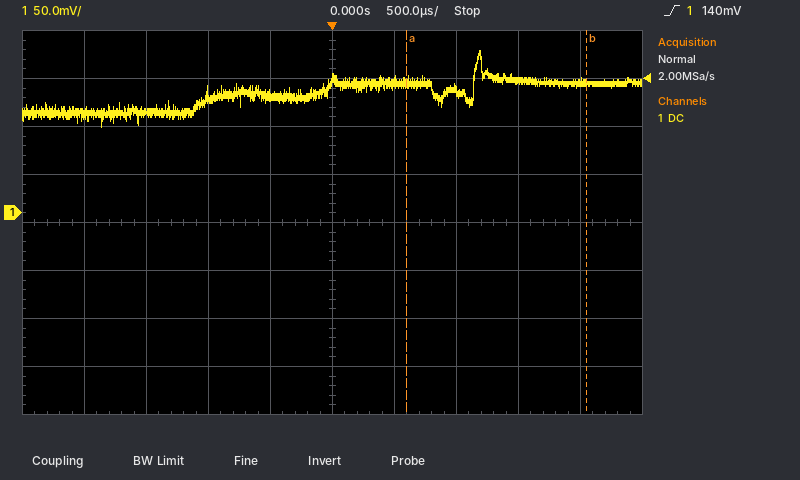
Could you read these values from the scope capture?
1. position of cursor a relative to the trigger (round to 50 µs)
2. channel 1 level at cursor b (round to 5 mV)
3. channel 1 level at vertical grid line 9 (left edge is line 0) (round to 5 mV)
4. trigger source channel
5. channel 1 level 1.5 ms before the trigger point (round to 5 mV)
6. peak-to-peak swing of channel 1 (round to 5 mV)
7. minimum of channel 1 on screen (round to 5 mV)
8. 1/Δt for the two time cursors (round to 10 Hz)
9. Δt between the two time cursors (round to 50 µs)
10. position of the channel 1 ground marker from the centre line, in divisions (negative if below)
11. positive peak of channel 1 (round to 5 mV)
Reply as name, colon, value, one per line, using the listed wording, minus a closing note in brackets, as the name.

position of cursor a relative to the trigger: +600 µs
channel 1 level at cursor b: 135 mV
channel 1 level at vertical grid line 9 (left edge is line 0): 135 mV
trigger source channel: channel 1
channel 1 level 1.5 ms before the trigger point: 105 mV
peak-to-peak swing of channel 1: 80 mV
minimum of channel 1 on screen: 90 mV
1/Δt for the two time cursors: 690 Hz
Δt between the two time cursors: 1.45 ms
position of the channel 1 ground marker from the centre line, in divisions: +0.2 div
positive peak of channel 1: 170 mV
